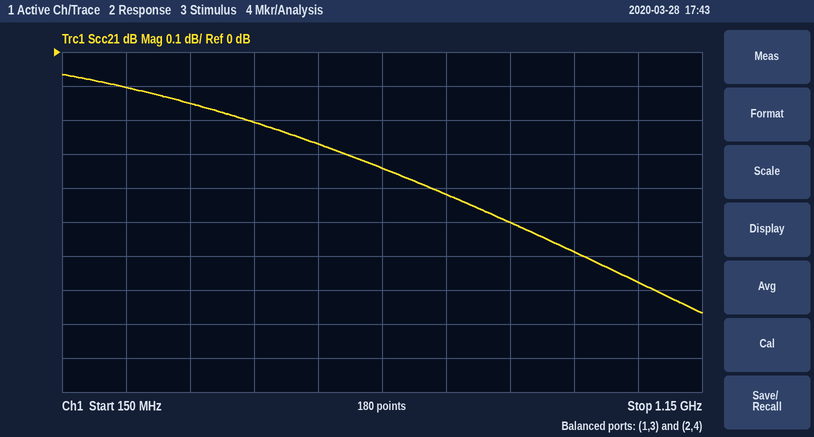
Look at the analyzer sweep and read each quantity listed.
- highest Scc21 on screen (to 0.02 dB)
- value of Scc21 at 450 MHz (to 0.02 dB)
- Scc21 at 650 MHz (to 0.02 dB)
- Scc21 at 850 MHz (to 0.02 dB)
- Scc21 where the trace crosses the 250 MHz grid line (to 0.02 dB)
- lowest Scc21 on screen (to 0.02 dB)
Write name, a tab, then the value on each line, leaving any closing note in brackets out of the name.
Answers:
highest Scc21 on screen	-0.06 dB
value of Scc21 at 450 MHz	-0.20 dB
Scc21 at 650 MHz	-0.34 dB
Scc21 at 850 MHz	-0.50 dB
Scc21 where the trace crosses the 250 MHz grid line	-0.10 dB
lowest Scc21 on screen	-0.76 dB
